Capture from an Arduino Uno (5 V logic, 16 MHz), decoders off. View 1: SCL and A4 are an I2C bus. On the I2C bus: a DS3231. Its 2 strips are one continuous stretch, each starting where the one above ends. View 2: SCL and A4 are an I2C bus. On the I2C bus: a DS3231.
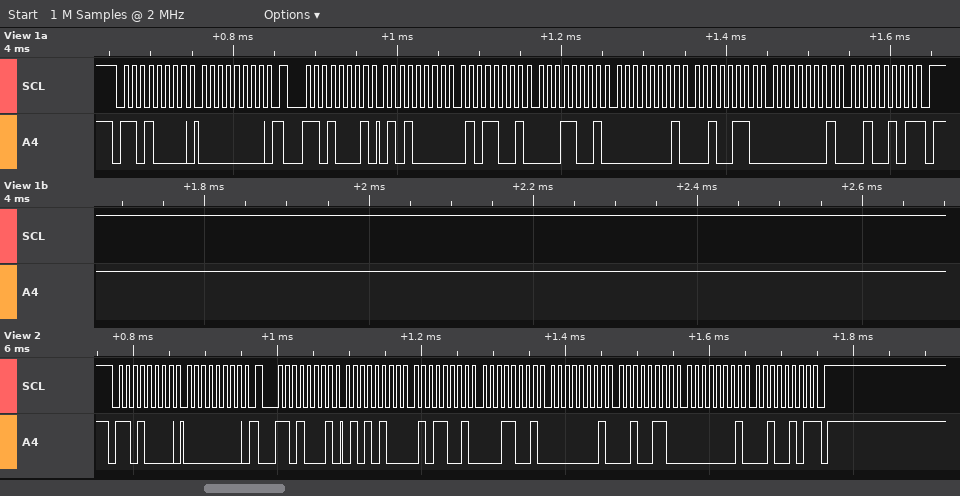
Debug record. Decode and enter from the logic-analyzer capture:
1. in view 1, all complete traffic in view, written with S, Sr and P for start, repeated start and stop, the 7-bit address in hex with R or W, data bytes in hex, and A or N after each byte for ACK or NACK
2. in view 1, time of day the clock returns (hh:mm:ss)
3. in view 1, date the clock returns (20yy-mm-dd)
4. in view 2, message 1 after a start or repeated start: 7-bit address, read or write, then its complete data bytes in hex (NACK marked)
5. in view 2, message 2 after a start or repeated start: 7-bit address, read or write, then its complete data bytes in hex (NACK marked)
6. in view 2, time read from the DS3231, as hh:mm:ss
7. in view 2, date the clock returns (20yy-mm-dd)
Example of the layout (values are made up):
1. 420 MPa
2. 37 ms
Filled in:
1. S 68W A 00 A Sr 68R A 50 A 59 A 19 A 01 A 26 A 01 A 25 N P
2. 19:59:50
3. 2025-01-26
4. 0x68 write: 00
5. 0x68 read: 54 59 19 01 26 01 25 NACK
6. 19:59:54
7. 2025-01-26
